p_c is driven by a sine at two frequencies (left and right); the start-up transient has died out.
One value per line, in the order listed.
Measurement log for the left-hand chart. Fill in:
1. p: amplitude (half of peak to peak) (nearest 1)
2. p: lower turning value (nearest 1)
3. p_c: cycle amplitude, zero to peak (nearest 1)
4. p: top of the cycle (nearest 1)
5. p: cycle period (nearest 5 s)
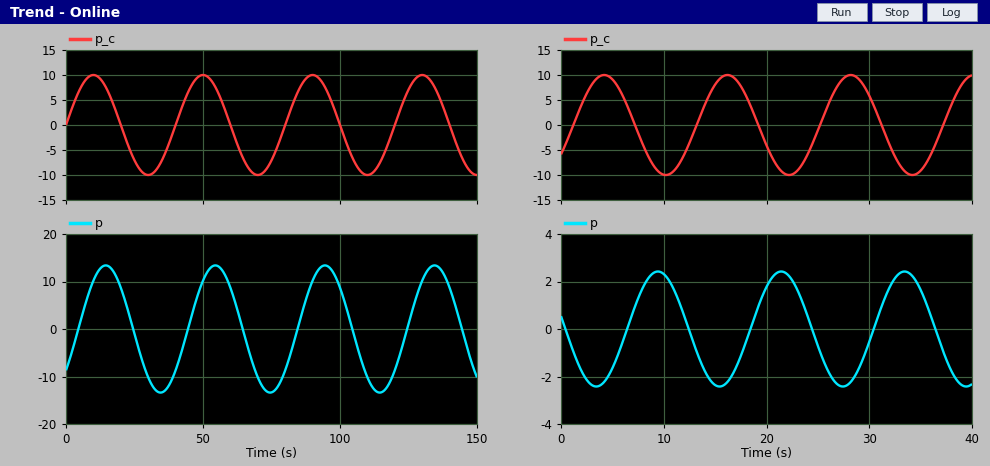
13
-13
10
13
40 s
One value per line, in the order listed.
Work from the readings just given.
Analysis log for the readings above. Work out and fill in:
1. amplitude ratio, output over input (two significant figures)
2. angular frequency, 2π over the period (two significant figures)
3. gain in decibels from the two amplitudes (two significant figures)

1.3
0.16 rad/s
2.3 dB
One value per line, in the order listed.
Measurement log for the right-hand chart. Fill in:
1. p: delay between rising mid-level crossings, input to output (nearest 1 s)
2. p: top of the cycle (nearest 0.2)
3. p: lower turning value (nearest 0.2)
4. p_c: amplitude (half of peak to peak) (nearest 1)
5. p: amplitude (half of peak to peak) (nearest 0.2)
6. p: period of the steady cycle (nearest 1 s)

5 s
2.4
-2.4
10
2.4
12 s
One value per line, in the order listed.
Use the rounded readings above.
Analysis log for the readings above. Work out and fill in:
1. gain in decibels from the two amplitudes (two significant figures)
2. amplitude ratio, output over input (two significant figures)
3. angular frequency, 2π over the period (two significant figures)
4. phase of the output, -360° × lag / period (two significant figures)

-12 dB
0.24
0.52 rad/s
-150°
